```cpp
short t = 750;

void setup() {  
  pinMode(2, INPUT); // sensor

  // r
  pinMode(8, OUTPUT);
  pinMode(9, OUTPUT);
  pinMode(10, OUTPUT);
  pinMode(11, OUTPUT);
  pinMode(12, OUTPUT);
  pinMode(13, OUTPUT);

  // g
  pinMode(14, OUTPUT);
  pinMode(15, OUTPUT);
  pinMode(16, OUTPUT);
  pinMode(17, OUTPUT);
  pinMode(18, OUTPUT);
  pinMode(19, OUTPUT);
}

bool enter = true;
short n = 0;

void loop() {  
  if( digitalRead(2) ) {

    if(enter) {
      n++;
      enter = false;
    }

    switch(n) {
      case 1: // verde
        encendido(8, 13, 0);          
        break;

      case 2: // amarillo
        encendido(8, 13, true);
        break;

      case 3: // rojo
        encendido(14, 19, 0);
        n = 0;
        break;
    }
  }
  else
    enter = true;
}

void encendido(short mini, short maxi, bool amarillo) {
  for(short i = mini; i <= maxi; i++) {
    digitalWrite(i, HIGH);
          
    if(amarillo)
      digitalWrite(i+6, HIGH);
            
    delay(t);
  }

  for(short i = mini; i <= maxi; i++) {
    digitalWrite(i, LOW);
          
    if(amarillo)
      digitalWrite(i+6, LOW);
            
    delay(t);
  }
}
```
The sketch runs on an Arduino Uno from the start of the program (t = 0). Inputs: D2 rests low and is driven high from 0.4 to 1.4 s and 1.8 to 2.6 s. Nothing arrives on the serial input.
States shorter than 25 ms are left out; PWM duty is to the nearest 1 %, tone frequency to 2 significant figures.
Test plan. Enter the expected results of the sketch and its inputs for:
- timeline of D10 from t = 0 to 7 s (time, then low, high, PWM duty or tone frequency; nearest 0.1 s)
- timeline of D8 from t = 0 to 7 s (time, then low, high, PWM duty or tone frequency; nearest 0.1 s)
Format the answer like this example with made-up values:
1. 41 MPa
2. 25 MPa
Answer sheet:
1. 0 s low; 1.9 s high; 6.4 s low
2. 0 s low; 0.4 s high; 4.9 s low
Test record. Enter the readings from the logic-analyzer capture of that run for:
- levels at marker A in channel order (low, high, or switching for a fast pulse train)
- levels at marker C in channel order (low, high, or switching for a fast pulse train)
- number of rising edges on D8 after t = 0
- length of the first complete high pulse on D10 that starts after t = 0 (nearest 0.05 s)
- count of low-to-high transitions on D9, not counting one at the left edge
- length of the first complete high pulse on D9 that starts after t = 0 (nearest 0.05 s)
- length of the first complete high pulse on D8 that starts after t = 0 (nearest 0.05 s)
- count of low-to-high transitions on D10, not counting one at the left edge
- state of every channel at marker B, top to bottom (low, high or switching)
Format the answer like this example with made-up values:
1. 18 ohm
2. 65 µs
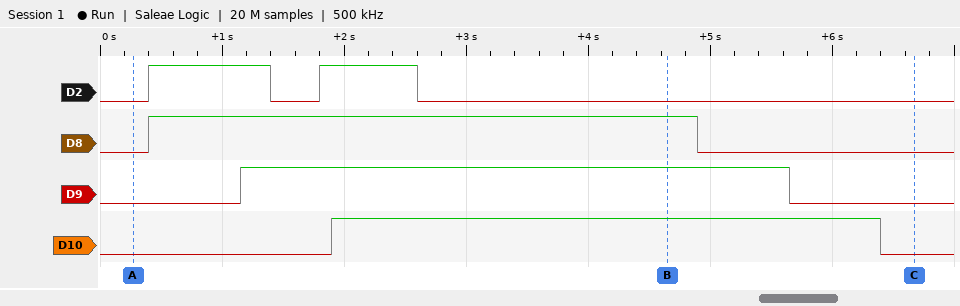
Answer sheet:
1. D2 low, D8 low, D9 low, D10 low
2. D2 low, D8 low, D9 low, D10 low
3. 1
4. 4.50 s
5. 1
6. 4.50 s
7. 4.50 s
8. 1
9. D2 low, D8 high, D9 high, D10 high
